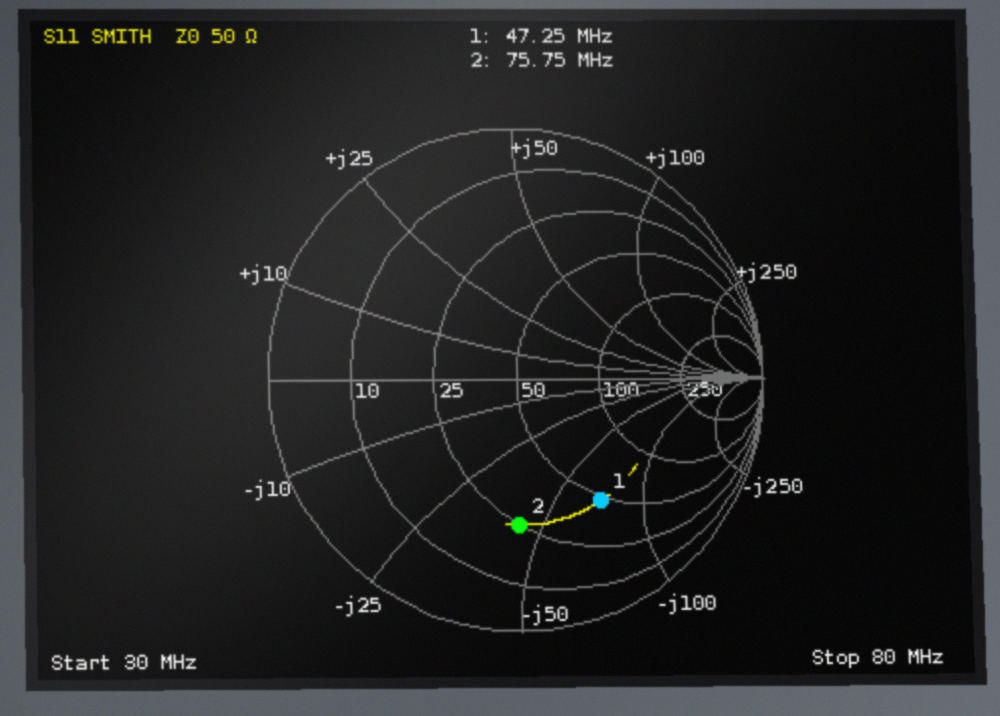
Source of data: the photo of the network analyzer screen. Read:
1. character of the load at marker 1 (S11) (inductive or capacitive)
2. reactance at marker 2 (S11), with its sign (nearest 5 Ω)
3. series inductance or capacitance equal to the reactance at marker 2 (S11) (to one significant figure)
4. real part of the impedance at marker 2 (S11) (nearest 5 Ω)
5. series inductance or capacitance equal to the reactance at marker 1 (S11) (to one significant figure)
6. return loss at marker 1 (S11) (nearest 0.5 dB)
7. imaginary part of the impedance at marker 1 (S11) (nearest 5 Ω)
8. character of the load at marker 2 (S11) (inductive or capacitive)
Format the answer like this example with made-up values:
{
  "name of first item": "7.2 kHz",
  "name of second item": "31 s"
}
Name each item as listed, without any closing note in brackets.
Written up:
{
  "character of the load at marker 1 (S11)": "capacitive",
  "reactance at marker 2 (S11), with its sign": "-45 Ω",
  "series inductance or capacitance equal to the reactance at marker 2 (S11)": "50 pF",
  "real part of the impedance at marker 2 (S11)": "25 Ω",
  "series inductance or capacitance equal to the reactance at marker 1 (S11)": "50 pF",
  "return loss at marker 1 (S11)": "4.5 dB",
  "imaginary part of the impedance at marker 1 (S11)": "-70 Ω",
  "character of the load at marker 2 (S11)": "capacitive"
}
